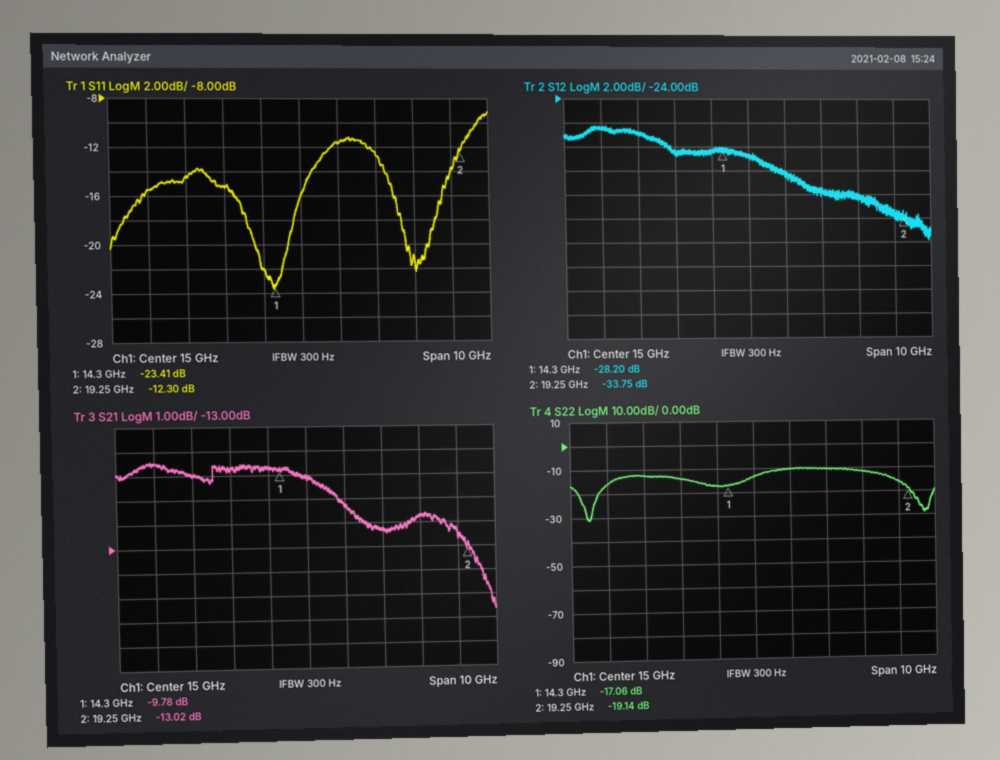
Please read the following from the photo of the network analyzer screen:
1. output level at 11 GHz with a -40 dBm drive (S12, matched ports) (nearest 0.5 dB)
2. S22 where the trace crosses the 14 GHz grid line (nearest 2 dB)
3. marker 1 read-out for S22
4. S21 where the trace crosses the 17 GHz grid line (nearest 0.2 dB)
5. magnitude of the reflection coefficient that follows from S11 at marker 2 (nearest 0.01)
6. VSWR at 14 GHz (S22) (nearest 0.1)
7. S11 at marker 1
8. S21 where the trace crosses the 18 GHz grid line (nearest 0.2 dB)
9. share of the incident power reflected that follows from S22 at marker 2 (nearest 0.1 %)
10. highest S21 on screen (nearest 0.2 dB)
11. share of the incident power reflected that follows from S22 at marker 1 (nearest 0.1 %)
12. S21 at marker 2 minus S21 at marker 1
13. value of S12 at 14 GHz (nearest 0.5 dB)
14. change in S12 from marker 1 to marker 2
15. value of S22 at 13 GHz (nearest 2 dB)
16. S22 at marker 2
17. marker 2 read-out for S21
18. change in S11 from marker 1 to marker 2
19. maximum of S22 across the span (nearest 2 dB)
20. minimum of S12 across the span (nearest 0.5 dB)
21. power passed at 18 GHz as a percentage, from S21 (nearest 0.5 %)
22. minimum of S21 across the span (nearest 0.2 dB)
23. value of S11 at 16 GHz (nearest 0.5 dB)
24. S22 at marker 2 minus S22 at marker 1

-66.5 dBm
-18 dB
-17.06 dB
-12.2 dB
0.24
1.3
-23.41 dB
-11.8 dB
1.2 %
-9.4 dB
2.0 %
-3.24 dB
-28.5 dB
-5.55 dB
-14 dB
-19.14 dB
-13.02 dB
11.11 dB
-10 dB
-36.0 dB
6.5 %
-15.6 dB
-11.5 dB
-2.08 dB
